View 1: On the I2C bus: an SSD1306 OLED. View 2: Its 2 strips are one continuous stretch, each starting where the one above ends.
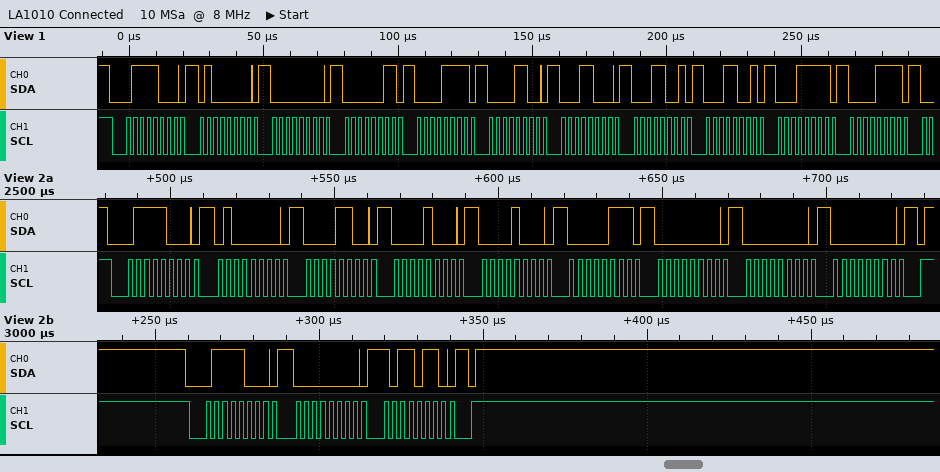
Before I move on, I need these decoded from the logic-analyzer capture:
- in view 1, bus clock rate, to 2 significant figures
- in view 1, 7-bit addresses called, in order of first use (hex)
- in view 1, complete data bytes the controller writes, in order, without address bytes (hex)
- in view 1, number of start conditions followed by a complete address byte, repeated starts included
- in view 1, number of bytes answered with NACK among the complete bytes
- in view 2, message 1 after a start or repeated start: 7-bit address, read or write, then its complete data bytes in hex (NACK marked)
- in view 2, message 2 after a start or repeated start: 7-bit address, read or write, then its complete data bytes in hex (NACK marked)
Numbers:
400 kHz
0x3C
40 00 03 0F 0C 18 19 19 1F 0F
1
0
0x3C write: 40 0C 08 08 07 00 00 00
0x3C write: 00 B6
